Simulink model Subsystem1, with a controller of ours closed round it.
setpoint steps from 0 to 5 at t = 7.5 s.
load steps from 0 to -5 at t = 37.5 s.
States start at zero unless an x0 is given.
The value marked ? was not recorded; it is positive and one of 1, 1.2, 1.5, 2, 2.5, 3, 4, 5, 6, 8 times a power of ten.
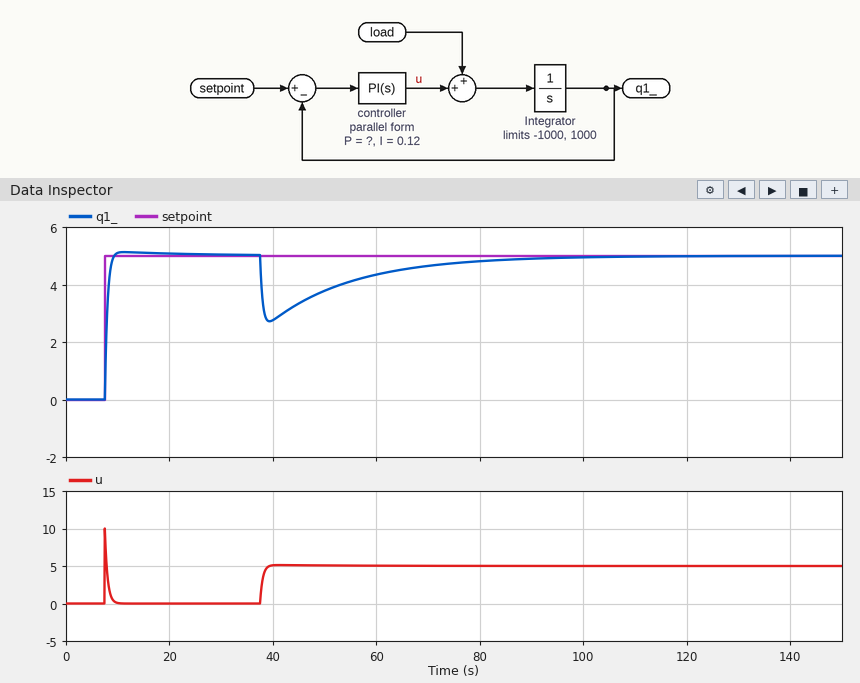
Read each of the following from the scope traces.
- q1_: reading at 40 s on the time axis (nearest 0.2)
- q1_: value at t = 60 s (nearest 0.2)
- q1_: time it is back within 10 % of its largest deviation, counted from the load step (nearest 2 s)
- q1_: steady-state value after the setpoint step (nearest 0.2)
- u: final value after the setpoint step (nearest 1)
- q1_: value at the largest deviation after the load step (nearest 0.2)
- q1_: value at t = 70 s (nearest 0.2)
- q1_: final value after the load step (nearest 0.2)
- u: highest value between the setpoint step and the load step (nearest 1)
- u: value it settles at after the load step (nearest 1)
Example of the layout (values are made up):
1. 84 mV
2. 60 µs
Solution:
1. 2.8
2. 4.4
3. 40 s
4. 5.0
5. 0
6. 2.8
7. 4.6
8. 5.0
9. 10
10. 5
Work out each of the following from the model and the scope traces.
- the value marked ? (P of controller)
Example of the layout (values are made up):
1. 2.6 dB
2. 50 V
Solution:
1. 2
